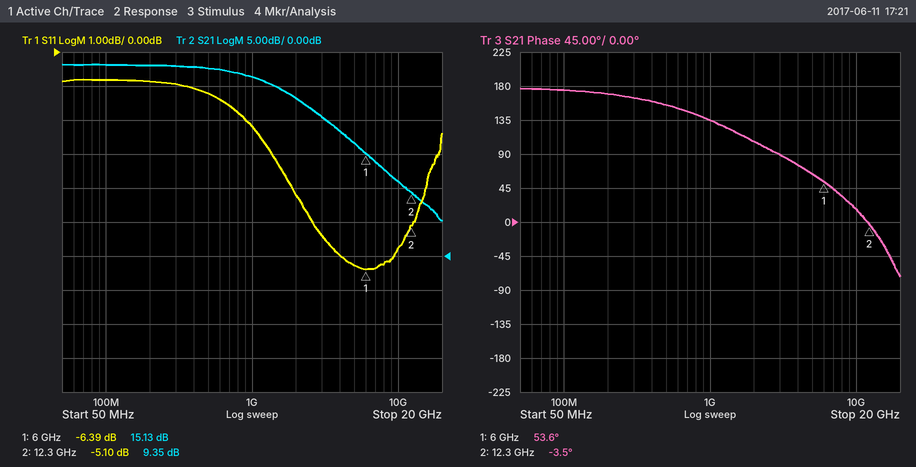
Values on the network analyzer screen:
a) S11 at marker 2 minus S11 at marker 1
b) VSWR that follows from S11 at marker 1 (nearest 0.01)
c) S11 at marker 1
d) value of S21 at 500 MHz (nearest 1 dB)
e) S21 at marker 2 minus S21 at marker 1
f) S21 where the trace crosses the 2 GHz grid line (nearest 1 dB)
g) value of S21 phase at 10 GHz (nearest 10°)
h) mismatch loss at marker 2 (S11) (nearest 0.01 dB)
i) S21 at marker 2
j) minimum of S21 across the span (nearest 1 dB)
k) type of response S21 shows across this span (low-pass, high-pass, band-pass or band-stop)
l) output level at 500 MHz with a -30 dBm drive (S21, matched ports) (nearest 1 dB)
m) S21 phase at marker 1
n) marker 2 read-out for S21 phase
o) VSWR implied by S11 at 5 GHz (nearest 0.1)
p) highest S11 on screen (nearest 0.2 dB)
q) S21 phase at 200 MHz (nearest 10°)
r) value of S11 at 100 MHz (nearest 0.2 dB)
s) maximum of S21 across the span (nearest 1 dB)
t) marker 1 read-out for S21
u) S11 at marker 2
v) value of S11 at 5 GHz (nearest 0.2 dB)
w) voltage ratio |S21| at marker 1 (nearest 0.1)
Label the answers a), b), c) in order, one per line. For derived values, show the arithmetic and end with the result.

a) -5.1 − (-6.39) = 1.29 dB
b) (1 + 0.4792)/(1 − 0.4792) ≈ 2.84
c) -6.39 dB
d) 28 dB
e) 9.35 − (15.13) = -5.78 dB
f) 23 dB
g) 20°
h) −10 log10(1 − 10^(-5.1/10)) ≈ 1.61 dB
i) 9.35 dB
j) 5 dB
k) low-pass
l) -30 dBm + (28 dB) = -2 dBm
m) 53.6°
n) -3.5°
o) |Γ| = 10^(-6.2/20) = 0.4898; VSWR = (1 + 0.4898)/(1 − 0.4898) ≈ 2.9
p) -0.8 dB
q) 170°
r) -0.8 dB
s) 28 dB
t) 15.13 dB
u) -5.10 dB
v) -6.2 dB
w) 10^(15.13/20) ≈ 5.7
